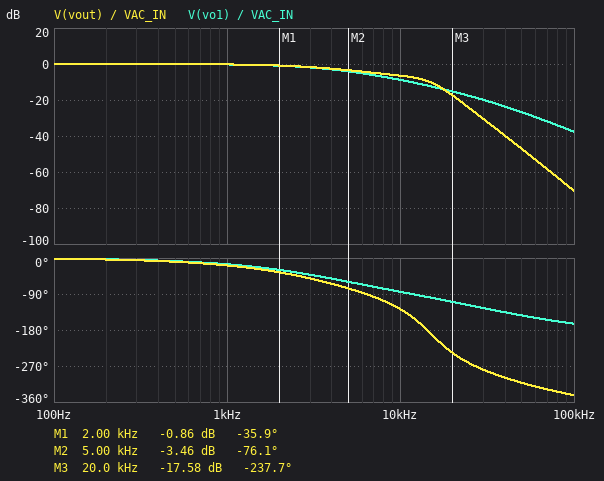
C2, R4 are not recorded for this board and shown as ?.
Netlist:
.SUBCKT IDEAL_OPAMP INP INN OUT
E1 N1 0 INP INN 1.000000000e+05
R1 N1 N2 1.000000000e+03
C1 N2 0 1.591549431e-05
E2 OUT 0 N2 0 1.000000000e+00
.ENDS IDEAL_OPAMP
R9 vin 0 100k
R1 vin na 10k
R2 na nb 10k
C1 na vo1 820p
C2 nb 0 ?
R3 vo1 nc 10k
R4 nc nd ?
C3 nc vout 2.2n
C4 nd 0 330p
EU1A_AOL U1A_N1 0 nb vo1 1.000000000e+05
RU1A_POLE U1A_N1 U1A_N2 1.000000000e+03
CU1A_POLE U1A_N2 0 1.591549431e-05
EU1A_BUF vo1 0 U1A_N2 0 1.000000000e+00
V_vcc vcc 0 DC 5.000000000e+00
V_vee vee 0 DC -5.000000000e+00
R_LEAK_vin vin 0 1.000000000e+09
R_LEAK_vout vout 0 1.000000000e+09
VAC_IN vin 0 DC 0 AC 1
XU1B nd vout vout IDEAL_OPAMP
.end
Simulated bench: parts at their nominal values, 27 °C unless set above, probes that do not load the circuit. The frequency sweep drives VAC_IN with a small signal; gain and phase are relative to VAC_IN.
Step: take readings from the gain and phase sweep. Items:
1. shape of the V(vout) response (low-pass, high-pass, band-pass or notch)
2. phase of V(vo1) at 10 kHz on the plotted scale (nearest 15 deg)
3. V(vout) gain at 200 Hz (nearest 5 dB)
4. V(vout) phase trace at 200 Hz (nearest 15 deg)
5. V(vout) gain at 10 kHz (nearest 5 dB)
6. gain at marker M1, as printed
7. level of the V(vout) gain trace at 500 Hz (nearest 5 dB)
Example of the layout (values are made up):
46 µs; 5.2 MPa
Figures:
low-pass; -90 deg; 0 dB; 0 deg; -5 dB; -0.86 dB; 0 dB
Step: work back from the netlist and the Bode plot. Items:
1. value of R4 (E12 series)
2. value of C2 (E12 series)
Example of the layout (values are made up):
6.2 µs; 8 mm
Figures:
15 kΩ; 2.2 nF
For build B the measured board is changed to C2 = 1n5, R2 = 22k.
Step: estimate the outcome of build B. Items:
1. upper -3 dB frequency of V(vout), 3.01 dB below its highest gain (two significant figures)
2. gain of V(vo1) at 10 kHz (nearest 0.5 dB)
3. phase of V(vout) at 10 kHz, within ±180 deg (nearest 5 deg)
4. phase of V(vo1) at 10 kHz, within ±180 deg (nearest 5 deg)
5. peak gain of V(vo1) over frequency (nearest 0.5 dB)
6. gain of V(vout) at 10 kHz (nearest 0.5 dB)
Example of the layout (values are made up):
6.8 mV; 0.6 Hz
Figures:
4.1 kHz; -9.5 dB; -135 deg; -90 deg; 0 dB; -7.0 dB
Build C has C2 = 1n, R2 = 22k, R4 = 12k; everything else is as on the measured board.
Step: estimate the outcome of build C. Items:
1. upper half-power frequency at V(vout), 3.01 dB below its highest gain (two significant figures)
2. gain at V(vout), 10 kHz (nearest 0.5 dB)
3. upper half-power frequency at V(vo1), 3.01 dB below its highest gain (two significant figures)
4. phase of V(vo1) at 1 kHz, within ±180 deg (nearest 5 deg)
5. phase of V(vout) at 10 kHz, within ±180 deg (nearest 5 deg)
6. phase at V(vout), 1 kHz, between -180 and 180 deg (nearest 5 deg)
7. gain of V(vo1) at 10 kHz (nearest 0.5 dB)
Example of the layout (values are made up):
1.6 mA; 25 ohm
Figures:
7.6 kHz; -4.0 dB; 6.0 kHz; -10 deg; -120 deg; -15 deg; -6.0 dB
